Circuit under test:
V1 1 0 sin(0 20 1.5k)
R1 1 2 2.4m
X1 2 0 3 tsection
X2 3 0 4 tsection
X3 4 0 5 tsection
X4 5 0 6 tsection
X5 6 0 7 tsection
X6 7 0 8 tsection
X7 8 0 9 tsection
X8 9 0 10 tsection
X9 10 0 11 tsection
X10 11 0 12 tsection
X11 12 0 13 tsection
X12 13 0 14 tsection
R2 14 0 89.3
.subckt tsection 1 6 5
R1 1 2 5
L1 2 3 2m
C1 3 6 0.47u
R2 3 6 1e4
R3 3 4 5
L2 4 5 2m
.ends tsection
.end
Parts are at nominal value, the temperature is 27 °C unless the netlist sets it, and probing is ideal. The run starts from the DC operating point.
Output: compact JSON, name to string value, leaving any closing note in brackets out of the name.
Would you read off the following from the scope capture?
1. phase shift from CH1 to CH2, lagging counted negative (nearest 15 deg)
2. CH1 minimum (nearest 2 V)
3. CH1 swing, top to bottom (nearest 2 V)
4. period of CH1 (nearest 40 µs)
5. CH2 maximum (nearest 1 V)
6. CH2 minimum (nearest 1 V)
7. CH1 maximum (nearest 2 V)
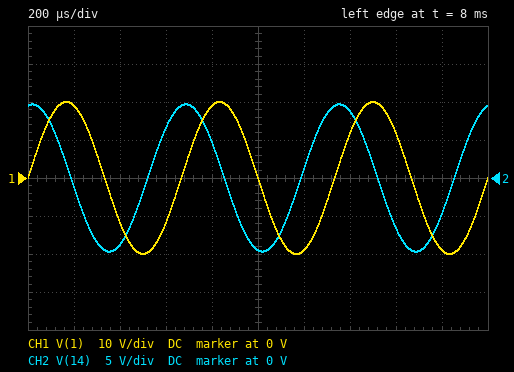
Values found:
{"phase shift from CH1 to CH2, lagging counted negative": "75 deg", "CH1 minimum": "-20 V", "CH1 swing, top to bottom": "40 V", "period of CH1": "680 µs", "CH2 maximum": "10 V", "CH2 minimum": "-10 V", "CH1 maximum": "20 V"}
